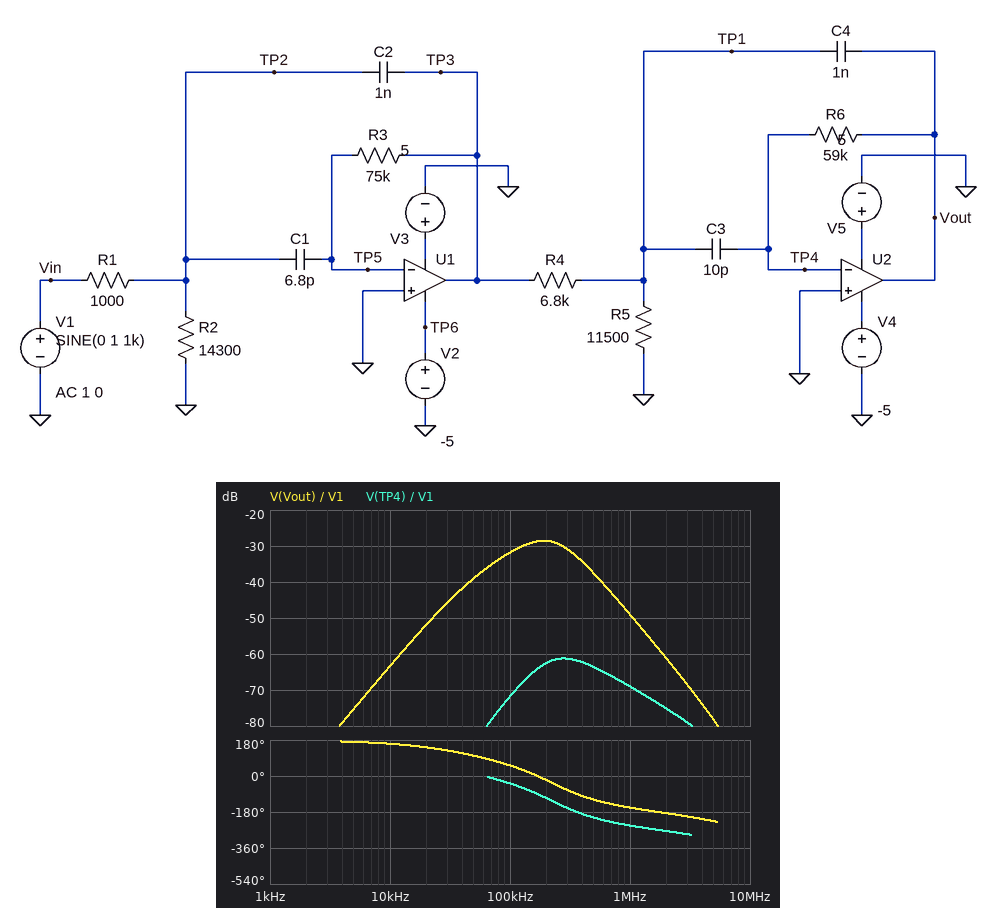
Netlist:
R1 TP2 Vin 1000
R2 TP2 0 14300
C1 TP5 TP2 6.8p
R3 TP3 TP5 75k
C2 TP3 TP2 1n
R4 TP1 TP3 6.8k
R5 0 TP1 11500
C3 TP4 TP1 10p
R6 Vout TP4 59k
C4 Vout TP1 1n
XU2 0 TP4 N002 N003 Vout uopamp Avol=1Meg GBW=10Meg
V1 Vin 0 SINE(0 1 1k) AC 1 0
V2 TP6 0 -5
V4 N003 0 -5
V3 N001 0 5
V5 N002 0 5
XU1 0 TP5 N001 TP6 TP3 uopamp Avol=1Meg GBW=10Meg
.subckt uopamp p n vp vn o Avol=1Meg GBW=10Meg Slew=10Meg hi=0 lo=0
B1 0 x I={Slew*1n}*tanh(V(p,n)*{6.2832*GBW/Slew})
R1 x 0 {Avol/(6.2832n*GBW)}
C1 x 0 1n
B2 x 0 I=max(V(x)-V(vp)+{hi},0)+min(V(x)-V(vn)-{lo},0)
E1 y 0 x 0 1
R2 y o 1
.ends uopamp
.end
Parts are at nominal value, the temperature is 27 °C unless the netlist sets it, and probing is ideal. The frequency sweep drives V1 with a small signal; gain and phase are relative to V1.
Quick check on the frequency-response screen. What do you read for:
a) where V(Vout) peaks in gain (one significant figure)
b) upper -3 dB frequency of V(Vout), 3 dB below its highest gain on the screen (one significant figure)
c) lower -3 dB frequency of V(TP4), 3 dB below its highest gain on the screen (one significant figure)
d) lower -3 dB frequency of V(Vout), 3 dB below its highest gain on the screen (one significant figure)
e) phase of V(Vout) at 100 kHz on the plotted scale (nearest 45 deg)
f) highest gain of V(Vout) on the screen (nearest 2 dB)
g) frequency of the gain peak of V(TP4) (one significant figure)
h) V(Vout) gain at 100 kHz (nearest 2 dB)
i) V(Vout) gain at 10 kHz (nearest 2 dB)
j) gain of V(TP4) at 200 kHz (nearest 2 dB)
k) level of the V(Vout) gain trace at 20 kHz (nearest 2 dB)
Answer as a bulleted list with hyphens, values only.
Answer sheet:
- 200 kHz
- 300 kHz
- 200 kHz
- 100 kHz
- 45 deg
- -28 dB
- 300 kHz
- -32 dB
- -64 dB
- -62 dB
- -52 dB
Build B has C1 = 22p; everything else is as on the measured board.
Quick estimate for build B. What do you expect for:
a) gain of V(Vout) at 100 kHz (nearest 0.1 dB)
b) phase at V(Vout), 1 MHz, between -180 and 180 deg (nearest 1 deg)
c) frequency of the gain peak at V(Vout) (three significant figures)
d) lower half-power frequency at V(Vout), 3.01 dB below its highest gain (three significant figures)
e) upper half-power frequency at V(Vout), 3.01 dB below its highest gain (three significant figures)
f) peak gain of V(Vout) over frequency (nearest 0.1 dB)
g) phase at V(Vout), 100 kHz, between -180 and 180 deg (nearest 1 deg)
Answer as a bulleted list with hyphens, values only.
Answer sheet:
- -18.6 dB
- -170 deg
- 125 kHz
- 87.0 kHz
- 175 kHz
- -17.3 dB
- 31 deg
